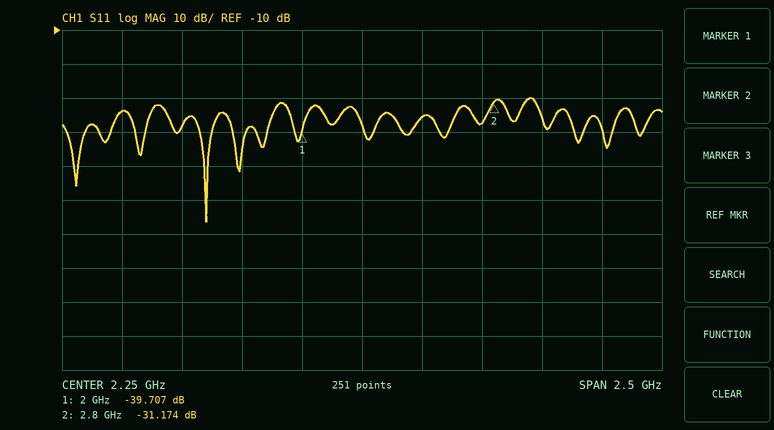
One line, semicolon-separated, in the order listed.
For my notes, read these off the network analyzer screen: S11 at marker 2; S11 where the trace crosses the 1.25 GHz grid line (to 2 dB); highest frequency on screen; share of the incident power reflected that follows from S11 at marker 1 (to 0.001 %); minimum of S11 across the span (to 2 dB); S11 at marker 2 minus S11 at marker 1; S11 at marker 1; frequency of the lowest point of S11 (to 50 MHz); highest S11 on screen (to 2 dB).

-31.174 dB; -34 dB; 3.5 GHz; 0.011 %; -66 dB; 8.533 dB; -39.707 dB; 1.60 GHz; -30 dB
